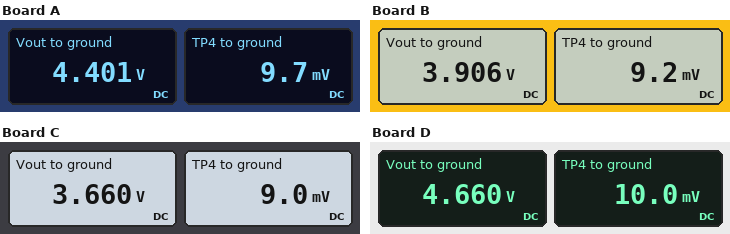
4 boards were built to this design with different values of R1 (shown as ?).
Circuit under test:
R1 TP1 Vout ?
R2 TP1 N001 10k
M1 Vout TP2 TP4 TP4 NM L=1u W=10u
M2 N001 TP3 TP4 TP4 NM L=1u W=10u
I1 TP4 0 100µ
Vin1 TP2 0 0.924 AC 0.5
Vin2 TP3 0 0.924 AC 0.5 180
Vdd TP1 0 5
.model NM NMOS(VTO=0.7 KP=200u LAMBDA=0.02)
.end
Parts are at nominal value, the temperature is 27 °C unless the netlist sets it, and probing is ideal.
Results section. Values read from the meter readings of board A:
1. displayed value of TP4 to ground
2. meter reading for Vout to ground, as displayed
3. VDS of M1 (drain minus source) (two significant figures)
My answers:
9.7 mV
4.401 V
4.4 V
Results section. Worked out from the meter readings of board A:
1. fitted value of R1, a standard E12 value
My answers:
12 kΩ
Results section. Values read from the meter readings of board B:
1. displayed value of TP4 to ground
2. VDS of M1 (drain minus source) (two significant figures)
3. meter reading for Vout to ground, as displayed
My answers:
9.2 mV
3.9 V
3.906 V
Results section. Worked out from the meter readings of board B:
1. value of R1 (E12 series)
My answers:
22 kΩ
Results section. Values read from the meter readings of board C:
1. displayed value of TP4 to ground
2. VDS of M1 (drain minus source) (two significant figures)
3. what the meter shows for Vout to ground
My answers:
9.0 mV
3.7 V
3.660 V
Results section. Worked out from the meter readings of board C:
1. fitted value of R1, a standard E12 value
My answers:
27 kΩ
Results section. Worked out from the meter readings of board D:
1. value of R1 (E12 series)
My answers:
6.8 kΩ
